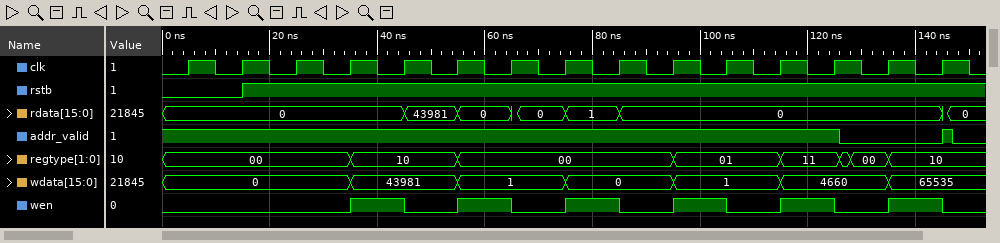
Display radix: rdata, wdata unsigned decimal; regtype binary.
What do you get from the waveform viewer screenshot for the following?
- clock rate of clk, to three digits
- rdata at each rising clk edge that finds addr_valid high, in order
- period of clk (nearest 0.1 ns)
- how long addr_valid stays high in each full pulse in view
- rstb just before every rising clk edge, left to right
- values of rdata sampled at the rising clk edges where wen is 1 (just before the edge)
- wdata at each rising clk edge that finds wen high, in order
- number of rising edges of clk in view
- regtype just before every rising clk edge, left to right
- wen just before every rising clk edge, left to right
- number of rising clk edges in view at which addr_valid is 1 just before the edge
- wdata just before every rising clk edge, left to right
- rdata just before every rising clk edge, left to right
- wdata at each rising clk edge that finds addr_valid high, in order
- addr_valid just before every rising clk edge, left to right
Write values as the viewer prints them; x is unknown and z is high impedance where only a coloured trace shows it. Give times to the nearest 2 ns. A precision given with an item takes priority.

100 MHz
0, 0, 0, 0, 0, 43981, 0, 0, 1, 0, 0, 0, 0
10 ns
2 ns
0 0 1 1 1 1 1 1 1 1 1 1 1 1 1
0, 0, 1, 0, 0, 0
43981, 1, 0, 1, 4660, 65535
15
00, 00, 00, 00, 10, 10, 00, 00, 00, 00, 01, 01, 11, 00, 10
0 0 0 0 1 0 1 0 1 0 1 0 1 0 1
13
0, 0, 0, 0, 43981, 43981, 1, 1, 0, 0, 1, 1, 4660, 4660, 65535
0, 0, 0, 0, 0, 43981, 0, 0, 1, 0, 0, 0, 0, 0, 0
0, 0, 0, 0, 43981, 43981, 1, 1, 0, 0, 1, 1, 4660
1 1 1 1 1 1 1 1 1 1 1 1 1 0 0
